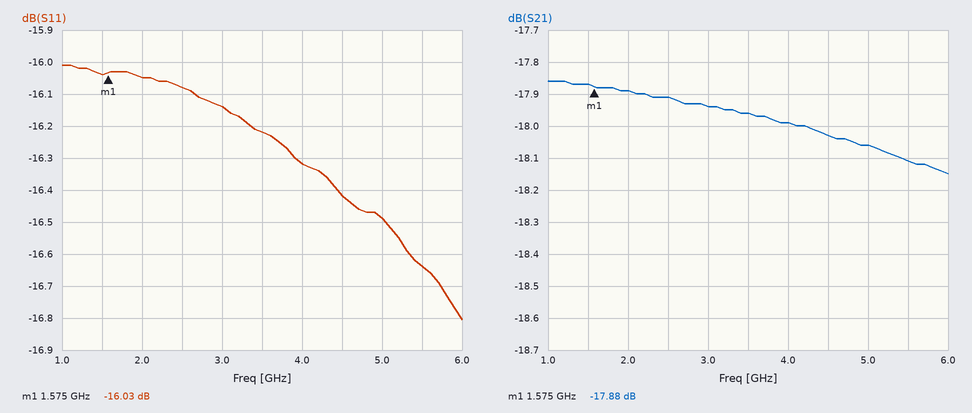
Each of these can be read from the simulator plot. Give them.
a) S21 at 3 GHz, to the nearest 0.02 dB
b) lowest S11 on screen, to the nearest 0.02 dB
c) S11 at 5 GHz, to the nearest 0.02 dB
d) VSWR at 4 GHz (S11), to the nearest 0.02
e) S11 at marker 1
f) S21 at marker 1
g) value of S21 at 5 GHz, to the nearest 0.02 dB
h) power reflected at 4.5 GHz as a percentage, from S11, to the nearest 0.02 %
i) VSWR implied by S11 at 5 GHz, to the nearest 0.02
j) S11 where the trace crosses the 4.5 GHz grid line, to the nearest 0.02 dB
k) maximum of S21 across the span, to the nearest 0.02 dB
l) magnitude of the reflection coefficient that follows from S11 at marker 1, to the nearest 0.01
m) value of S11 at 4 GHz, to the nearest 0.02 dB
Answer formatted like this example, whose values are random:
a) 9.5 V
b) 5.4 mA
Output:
a) -17.94 dB
b) -16.80 dB
c) -16.48 dB
d) 1.36
e) -16.03 dB
f) -17.88 dB
g) -18.06 dB
h) 2.28 %
i) 1.36
j) -16.42 dB
k) -17.86 dB
l) 0.16
m) -16.32 dB
